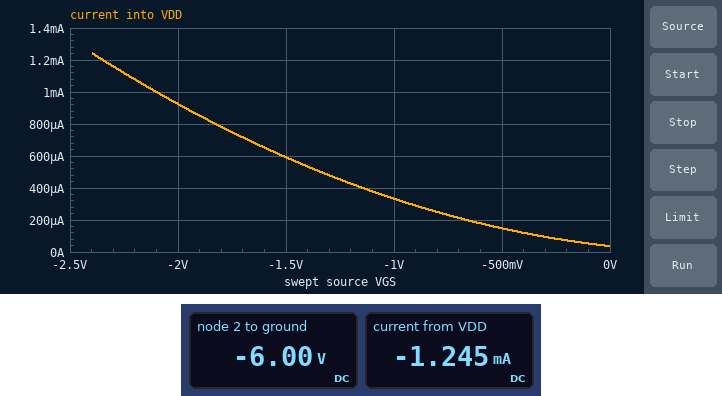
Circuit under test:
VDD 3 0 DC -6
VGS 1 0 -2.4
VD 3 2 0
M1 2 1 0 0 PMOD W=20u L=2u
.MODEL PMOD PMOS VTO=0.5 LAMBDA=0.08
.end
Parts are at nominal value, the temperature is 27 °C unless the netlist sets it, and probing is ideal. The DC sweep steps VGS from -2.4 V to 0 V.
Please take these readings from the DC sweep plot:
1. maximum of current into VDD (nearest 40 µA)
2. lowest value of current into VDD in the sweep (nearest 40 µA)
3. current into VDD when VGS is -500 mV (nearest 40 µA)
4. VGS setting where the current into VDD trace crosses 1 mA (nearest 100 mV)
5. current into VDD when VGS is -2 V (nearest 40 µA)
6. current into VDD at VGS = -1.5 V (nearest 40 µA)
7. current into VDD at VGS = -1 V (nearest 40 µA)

1.24 mA
40 µA
160 µA
-2.1 V
920 µA
600 µA
320 µA
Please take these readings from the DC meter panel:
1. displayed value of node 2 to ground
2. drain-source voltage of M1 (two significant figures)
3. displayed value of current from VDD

-6.00 V
-6.0 V
-1.245 mA
